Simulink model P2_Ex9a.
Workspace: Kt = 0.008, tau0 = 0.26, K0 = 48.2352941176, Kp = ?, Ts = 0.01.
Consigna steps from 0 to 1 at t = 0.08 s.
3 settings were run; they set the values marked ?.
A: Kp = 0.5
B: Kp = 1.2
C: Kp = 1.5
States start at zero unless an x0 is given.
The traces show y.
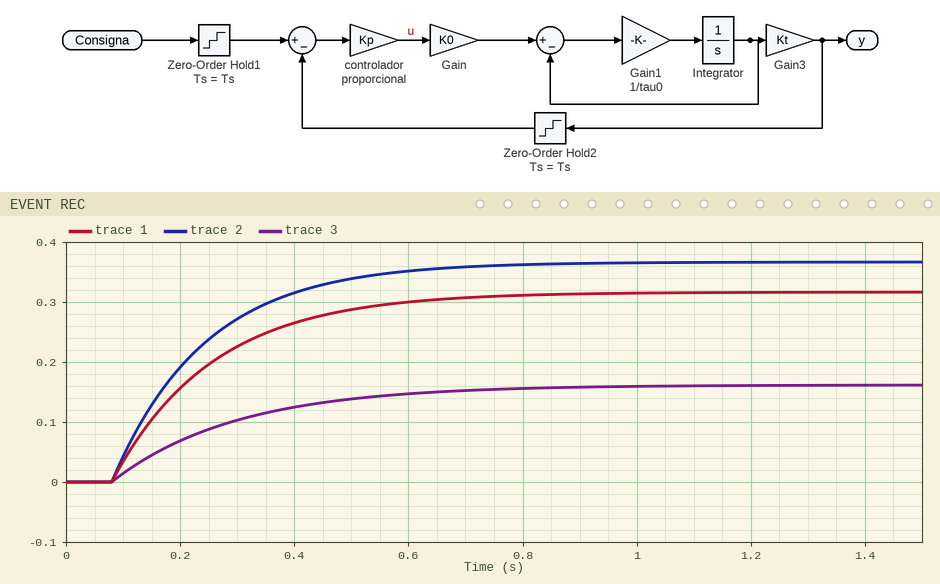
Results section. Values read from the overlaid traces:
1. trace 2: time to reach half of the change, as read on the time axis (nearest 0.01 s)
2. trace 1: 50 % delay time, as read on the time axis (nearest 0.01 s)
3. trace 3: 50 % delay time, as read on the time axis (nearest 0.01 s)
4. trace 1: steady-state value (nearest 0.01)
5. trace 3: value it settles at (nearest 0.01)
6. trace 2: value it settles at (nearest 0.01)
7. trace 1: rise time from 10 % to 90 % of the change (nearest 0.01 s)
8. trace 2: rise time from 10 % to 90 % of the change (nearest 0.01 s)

0.19 s
0.20 s
0.23 s
0.32
0.16
0.37
0.39 s
0.36 s
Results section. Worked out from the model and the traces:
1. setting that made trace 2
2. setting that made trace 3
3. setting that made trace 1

C
A
B
